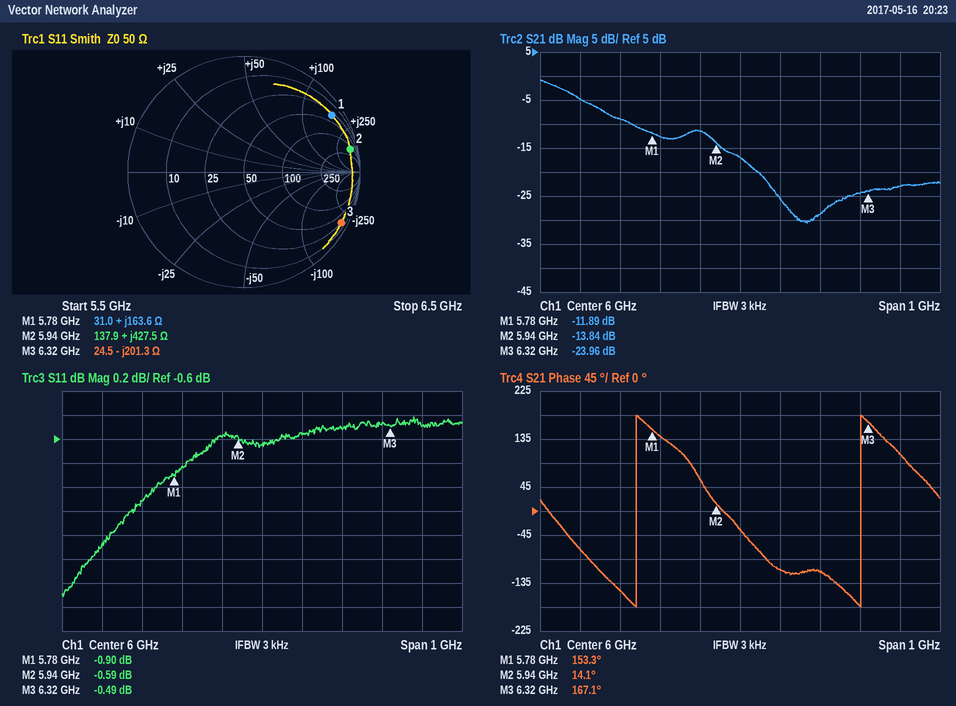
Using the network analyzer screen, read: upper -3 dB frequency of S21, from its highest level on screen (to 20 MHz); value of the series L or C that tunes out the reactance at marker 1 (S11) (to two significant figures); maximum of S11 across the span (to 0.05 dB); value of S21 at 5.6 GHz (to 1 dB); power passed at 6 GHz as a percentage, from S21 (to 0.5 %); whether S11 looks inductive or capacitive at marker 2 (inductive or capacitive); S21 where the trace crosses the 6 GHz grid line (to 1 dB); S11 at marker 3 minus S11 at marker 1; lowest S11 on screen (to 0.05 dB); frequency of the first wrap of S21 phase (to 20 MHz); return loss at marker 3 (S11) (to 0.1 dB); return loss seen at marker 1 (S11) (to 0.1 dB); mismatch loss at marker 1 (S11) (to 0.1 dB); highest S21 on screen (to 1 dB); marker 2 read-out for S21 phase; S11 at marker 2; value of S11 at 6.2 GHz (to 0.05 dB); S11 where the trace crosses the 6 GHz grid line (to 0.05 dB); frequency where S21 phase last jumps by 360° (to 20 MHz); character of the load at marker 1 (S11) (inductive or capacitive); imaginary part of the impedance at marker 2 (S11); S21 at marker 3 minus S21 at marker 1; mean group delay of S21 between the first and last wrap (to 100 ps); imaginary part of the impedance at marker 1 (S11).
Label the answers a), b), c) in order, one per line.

a) 5.58 GHz
b) 170 fF
c) -0.40 dB
d) -5 dB
e) 2.0 %
f) inductive
g) -17 dB
h) 0.41 dB
i) -1.90 dB
j) 5.74 GHz
k) 0.5 dB
l) 0.9 dB
m) 7.3 dB
n) -1 dB
o) 14.1°
p) -0.59 dB
q) -0.50 dB
r) -0.65 dB
s) 6.30 GHz
t) inductive
u) +427.5 Ω
v) -12.07 dB
w) 1.8 ns
x) +163.6 Ω
